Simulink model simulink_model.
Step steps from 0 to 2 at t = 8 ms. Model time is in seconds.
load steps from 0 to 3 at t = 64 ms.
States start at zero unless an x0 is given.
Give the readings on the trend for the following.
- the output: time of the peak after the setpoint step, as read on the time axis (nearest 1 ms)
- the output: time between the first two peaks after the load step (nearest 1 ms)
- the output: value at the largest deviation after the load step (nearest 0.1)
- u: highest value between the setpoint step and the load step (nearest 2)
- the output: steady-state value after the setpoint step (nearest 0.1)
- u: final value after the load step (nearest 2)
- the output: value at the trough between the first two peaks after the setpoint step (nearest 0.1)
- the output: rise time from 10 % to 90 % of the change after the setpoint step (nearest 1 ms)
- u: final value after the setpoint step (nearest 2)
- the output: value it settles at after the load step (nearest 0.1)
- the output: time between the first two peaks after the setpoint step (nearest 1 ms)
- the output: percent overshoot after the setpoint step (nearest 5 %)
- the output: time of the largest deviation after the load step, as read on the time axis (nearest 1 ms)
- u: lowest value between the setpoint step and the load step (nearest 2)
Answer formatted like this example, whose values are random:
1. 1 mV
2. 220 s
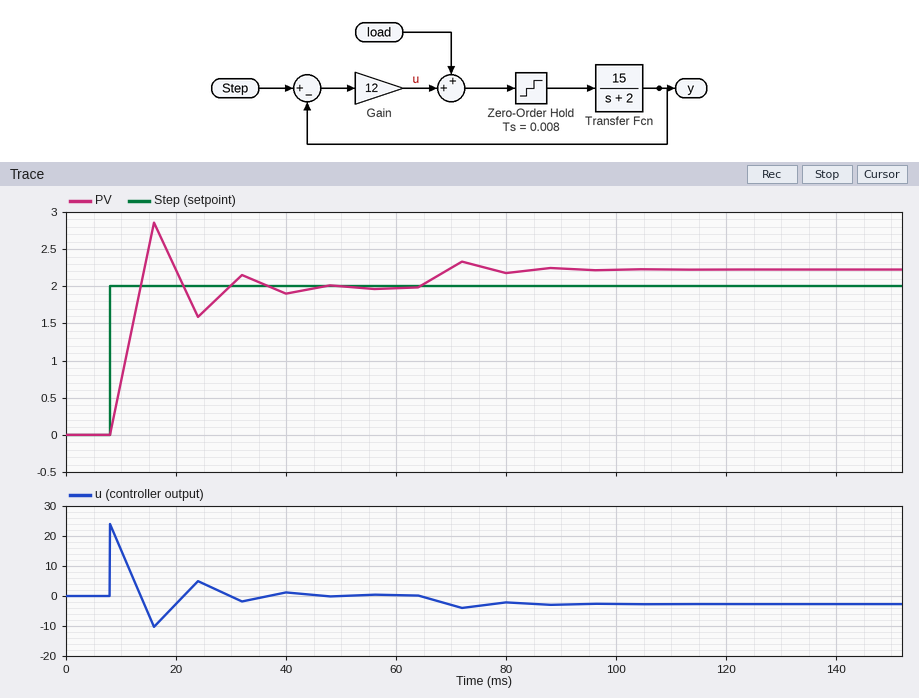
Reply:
1. 16 ms
2. 16 ms
3. 2.3
4. 24
5. 2.0
6. -2
7. 1.6
8. 4 ms
9. 0
10. 2.2
11. 16 ms
12. 45 %
13. 72 ms
14. -10
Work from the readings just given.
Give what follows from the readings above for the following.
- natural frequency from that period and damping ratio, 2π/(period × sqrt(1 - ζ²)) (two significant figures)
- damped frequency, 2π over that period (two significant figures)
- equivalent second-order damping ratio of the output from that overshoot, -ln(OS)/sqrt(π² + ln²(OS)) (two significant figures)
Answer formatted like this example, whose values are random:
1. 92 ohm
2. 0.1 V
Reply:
1. 0.41 rad/ms
2. 0.39 rad/ms
3. 0.25
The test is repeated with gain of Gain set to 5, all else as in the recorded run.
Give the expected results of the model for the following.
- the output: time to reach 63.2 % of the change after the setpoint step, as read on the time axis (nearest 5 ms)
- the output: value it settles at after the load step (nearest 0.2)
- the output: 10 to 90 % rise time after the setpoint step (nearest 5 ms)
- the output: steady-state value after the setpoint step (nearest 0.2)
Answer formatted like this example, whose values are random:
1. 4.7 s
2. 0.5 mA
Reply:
1. 15 ms
2. 2.6
3. 20 ms
4. 2.0
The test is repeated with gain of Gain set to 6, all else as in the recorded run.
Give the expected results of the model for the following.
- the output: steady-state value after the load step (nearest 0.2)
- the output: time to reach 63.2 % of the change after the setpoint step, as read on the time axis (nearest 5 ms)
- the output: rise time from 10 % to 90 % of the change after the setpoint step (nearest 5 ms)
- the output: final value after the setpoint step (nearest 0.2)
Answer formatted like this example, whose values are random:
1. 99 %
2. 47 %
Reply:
1. 2.4
2. 15 ms
3. 15 ms
4. 2.0
